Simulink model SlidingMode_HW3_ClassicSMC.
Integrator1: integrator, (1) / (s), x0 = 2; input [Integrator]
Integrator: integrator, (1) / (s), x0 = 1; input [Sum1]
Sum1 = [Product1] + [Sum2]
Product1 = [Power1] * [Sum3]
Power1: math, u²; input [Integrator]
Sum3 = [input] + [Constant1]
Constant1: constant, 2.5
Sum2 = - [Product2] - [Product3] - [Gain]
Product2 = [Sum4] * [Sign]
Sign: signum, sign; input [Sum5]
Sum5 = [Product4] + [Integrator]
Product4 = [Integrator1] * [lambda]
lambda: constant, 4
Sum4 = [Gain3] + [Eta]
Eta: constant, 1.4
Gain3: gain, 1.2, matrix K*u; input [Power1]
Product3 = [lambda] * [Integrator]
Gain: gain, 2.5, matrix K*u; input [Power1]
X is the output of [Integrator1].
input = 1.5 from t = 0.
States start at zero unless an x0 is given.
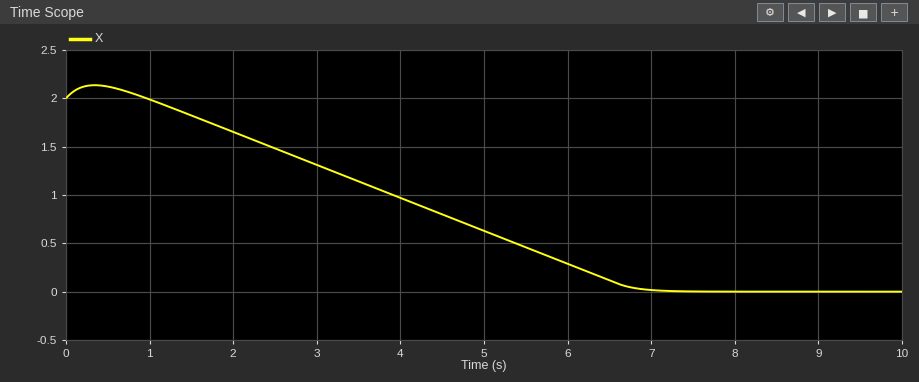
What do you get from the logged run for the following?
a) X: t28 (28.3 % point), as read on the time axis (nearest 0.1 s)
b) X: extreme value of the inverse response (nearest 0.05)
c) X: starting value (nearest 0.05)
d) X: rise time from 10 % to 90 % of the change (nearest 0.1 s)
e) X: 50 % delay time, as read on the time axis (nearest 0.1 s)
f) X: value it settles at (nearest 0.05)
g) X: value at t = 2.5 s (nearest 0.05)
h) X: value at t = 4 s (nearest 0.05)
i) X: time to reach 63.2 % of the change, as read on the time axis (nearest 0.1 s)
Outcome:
2.6 s
2.15
2.00
4.7 s
3.9 s
0.00
1.50
0.95
4.7 s
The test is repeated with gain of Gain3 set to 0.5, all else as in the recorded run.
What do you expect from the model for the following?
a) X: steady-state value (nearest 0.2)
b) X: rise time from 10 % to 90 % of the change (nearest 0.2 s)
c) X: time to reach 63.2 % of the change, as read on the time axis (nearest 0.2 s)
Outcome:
0.0
5.0 s
5.0 s
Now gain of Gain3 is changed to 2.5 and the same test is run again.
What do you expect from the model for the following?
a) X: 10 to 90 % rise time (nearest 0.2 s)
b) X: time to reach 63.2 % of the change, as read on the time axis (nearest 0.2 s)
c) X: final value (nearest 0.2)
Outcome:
4.2 s
4.2 s
0.0
